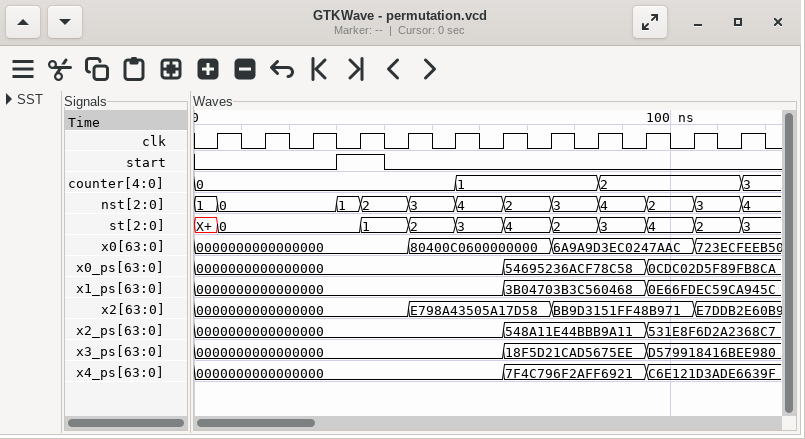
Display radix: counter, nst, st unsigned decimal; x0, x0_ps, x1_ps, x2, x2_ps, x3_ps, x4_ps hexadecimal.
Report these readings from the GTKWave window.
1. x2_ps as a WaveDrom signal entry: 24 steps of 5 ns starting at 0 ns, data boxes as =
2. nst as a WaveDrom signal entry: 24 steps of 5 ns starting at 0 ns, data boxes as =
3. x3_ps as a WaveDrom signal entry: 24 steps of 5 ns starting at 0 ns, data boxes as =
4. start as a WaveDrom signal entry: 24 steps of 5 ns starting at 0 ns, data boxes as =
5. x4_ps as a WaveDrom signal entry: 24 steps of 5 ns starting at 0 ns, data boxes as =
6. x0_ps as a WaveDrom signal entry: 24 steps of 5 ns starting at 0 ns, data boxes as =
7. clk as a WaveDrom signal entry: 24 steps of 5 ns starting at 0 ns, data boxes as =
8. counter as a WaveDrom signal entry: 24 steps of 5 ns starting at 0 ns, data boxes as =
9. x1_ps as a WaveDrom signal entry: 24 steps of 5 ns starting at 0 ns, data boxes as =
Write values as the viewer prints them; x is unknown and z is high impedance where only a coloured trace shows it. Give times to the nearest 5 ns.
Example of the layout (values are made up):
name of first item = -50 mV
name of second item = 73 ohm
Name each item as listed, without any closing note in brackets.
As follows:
x2_ps as a WaveDrom signal entry: 24 steps of 5 ns starting at 0 ns, data boxes as = = {name: 'x2_ps', wave: '=............=.....=....', data: '0000000000000000 548A11E44BBB9A11 531E8F6D2A2368C7'}
nst as a WaveDrom signal entry: 24 steps of 5 ns starting at 0 ns, data boxes as = = {name: 'nst', wave: '==....==.=.=.=.=.=.=.=.=', data: '1 0 1 2 3 4 2 3 4 2 3 4'}
x3_ps as a WaveDrom signal entry: 24 steps of 5 ns starting at 0 ns, data boxes as = = {name: 'x3_ps', wave: '=............=.....=....', data: '0000000000000000 18F5D21CAD5675EE D579918416BEE980'}
start as a WaveDrom signal entry: 24 steps of 5 ns starting at 0 ns, data boxes as = = {name: 'start', wave: '0.....1.0...............'}
x4_ps as a WaveDrom signal entry: 24 steps of 5 ns starting at 0 ns, data boxes as = = {name: 'x4_ps', wave: '=............=.....=....', data: '0000000000000000 7F4C796F2AFF6921 C6E121D3ADE6639F'}
x0_ps as a WaveDrom signal entry: 24 steps of 5 ns starting at 0 ns, data boxes as = = {name: 'x0_ps', wave: '=............=.....=....', data: '0000000000000000 54695236ACF78C58 0CDC02D5F89FB8CA'}
clk as a WaveDrom signal entry: 24 steps of 5 ns starting at 0 ns, data boxes as = = {name: 'clk', wave: '010101010101010101010101'}
counter as a WaveDrom signal entry: 24 steps of 5 ns starting at 0 ns, data boxes as = = {name: 'counter', wave: '=..........=.....=.....=', data: '0 1 2 3'}
x1_ps as a WaveDrom signal entry: 24 steps of 5 ns starting at 0 ns, data boxes as = = {name: 'x1_ps', wave: '=............=.....=....', data: '0000000000000000 3B04703B3C560468 0E66FDEC59CA945C'}
